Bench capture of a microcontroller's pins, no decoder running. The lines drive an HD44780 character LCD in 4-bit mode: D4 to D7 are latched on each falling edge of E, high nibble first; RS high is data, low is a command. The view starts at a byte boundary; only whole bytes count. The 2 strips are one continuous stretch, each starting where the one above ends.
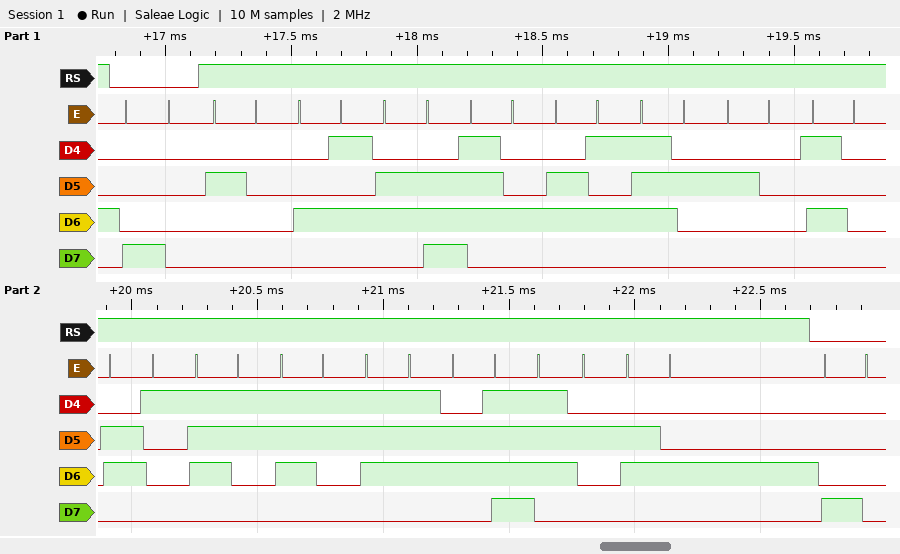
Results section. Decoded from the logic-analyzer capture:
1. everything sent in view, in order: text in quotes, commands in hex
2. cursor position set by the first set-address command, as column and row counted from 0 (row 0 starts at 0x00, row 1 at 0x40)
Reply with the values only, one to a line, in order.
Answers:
0x80 " Enter Password" 0x80
column 0, row 0
